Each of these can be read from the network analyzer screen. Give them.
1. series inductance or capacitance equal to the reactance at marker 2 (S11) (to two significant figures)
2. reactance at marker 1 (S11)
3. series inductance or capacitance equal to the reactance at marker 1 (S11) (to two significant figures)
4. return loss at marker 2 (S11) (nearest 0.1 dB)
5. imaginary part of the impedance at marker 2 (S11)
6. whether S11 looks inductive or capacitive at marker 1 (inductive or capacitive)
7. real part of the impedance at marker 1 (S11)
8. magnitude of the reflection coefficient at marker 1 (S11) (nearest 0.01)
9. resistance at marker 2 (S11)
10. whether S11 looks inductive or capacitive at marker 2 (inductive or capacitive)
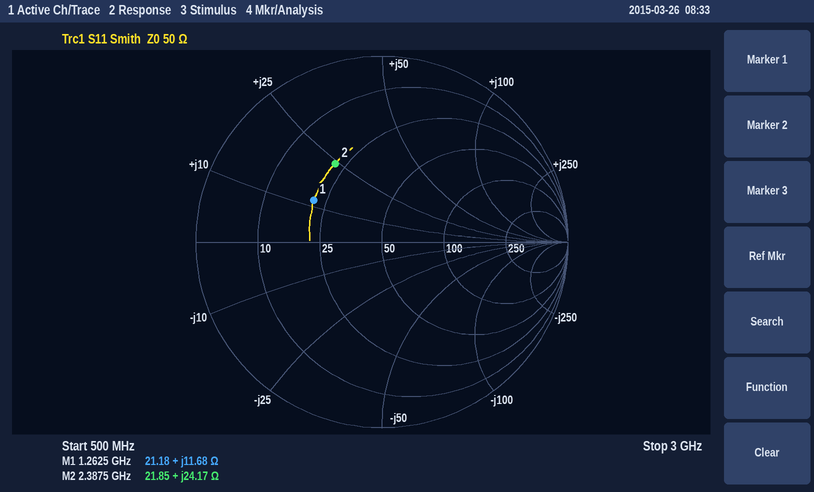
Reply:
1.6 nH
+11.68 Ω
1.5 nH
6.2 dB
+24.17 Ω
inductive
21.18 Ω
0.43
21.85 Ω
inductive
